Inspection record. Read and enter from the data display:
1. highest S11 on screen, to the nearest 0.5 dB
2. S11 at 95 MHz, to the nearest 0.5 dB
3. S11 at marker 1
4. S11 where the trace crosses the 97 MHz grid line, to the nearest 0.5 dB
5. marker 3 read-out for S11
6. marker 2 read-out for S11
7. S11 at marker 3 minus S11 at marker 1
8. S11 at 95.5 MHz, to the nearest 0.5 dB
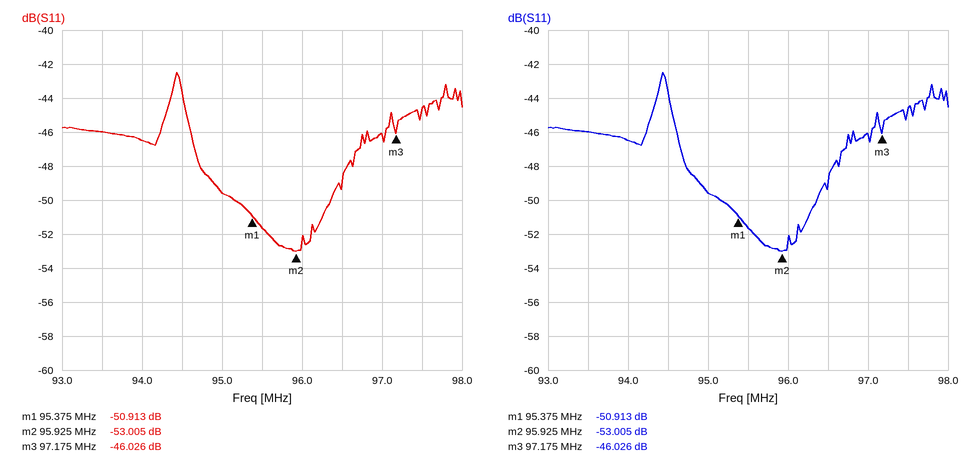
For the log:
-42.5 dB
-49.5 dB
-50.913 dB
-46.0 dB
-46.026 dB
-53.005 dB
4.887 dB
-51.5 dB
